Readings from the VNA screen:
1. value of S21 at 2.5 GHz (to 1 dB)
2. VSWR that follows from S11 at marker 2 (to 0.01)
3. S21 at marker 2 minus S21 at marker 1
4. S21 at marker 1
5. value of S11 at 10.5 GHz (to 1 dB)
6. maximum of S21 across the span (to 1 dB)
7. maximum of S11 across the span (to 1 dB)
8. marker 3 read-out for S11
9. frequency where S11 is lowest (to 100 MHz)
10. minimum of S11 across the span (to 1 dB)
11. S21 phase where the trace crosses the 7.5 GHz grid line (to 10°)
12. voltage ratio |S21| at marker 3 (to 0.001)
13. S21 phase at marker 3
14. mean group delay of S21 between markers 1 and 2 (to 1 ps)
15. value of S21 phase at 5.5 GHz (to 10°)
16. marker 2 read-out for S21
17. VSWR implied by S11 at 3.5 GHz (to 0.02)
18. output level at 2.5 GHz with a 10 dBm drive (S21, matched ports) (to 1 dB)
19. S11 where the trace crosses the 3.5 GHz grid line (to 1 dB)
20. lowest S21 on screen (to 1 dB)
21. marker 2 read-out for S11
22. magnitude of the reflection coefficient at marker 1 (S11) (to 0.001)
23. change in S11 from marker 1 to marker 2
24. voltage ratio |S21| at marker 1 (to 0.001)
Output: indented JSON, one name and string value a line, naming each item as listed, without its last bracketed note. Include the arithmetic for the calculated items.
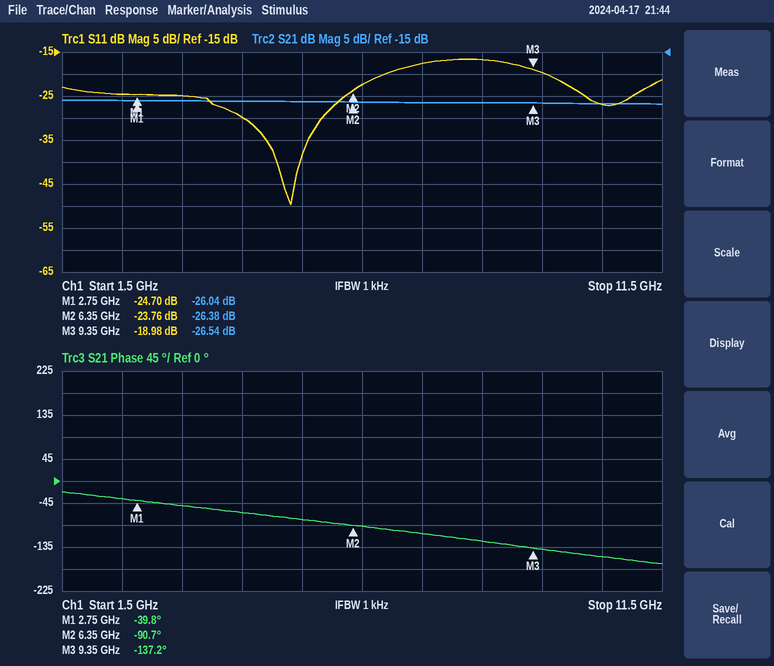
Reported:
{
  "value of S21 at 2.5 GHz": "-26 dB",
  "VSWR that follows from S11 at marker 2": "(1 + 0.0649)/(1 − 0.0649) ≈ 1.14",
  "S21 at marker 2 minus S21 at marker 1": "-26.38 − (-26.04) = -0.34 dB",
  "S21 at marker 1": "-26.04 dB",
  "value of S11 at 10.5 GHz": "-27 dB",
  "maximum of S21 across the span": "-26 dB",
  "maximum of S11 across the span": "-17 dB",
  "marker 3 read-out for S11": "-18.98 dB",
  "frequency where S11 is lowest": "5.3 GHz",
  "minimum of S11 across the span": "-50 dB",
  "S21 phase where the trace crosses the 7.5 GHz grid line": "-110°",
  "voltage ratio |S21| at marker 3": "10^(-26.54/20) ≈ 0.047",
  "S21 phase at marker 3": "-137.2°",
  "mean group delay of S21 between markers 1 and 2": "−(-90.7° − (-39.8°))/(360° × 3.6 GHz) ≈ 39 ps",
  "value of S21 phase at 5.5 GHz": "-80°",
  "marker 2 read-out for S21": "-26.38 dB",
  "VSWR implied by S11 at 3.5 GHz": "|Γ| = 10^(-25/20) = 0.0562; VSWR = (1 + 0.0562)/(1 − 0.0562) ≈ 1.12",
  "output level at 2.5 GHz with a 10 dBm drive (S21, matched ports)": "10 dBm + (-26 dB) = -16 dBm",
  "S11 where the trace crosses the 3.5 GHz grid line": "-25 dB",
  "lowest S21 on screen": "-27 dB",
  "marker 2 read-out for S11": "-23.76 dB",
  "magnitude of the reflection coefficient at marker 1 (S11)": "10^(-24.7/20) ≈ 0.058",
  "change in S11 from marker 1 to marker 2": "-23.76 − (-24.7) = 0.94 dB",
  "voltage ratio |S21| at marker 1": "10^(-26.04/20) ≈ 0.050"
}
